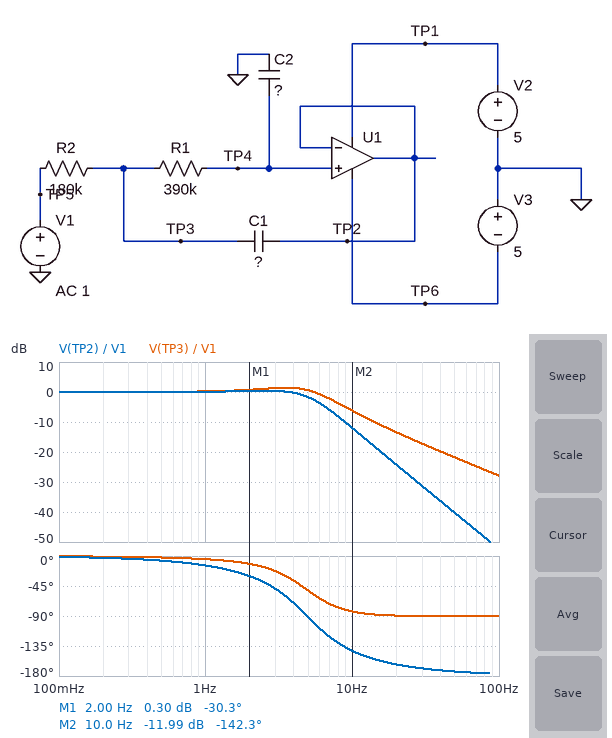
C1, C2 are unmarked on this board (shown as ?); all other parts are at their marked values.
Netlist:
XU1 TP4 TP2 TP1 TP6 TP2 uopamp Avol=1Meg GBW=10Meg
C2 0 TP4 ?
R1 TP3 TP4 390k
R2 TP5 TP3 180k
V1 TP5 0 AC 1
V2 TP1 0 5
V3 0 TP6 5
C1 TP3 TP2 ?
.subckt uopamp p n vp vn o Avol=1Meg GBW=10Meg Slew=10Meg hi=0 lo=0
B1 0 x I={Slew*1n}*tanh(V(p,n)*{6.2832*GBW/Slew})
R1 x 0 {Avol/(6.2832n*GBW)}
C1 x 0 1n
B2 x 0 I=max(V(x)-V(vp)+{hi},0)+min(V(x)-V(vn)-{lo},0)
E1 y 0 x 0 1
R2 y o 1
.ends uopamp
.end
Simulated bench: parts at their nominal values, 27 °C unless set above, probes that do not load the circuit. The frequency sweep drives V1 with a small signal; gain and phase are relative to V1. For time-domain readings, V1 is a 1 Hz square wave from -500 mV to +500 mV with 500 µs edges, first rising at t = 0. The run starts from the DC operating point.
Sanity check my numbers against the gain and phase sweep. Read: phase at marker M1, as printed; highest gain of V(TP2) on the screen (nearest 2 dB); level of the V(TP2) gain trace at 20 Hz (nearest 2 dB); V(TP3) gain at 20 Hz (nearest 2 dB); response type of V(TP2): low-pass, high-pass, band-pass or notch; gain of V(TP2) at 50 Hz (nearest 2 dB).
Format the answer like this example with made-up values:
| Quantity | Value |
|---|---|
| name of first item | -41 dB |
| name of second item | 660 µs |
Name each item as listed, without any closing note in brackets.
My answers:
| Quantity | Value |
|---|---|
| phase at marker M1, as printed | -30.3 deg |
| highest gain of V(TP2) on the screen | 0 dB |
| level of the V(TP2) gain trace at 20 Hz | -24 dB |
| V(TP3) gain at 20 Hz | -14 dB |
| response type of V(TP2): low-pass, high-pass, band-pass or notch | low-pass |
| gain of V(TP2) at 50 Hz | -40 dB |
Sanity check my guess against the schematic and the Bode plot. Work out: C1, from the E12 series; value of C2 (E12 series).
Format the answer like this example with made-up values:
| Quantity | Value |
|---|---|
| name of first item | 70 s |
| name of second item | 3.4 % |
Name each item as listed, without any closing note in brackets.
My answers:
| Quantity | Value |
|---|---|
| C1, from the E12 series | 220 nF |
| value of C2 | 68 nF |
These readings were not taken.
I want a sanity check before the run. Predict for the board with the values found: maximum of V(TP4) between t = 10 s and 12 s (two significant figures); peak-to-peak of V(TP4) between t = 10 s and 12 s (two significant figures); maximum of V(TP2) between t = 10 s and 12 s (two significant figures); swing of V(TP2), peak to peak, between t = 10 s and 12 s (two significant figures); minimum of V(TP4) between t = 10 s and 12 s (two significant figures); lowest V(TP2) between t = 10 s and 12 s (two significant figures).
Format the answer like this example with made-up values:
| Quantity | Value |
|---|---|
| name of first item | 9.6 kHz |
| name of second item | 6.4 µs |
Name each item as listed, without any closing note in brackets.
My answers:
| Quantity | Value |
|---|---|
| maximum of V(TP4) between t = 10 s and 12 s | 600 mV |
| peak-to-peak of V(TP4) between t = 10 s and 12 s | 1.2 V |
| maximum of V(TP2) between t = 10 s and 12 s | 600 mV |
| swing of V(TP2), peak to peak, between t = 10 s and 12 s | 1.2 V |
| minimum of V(TP4) between t = 10 s and 12 s | -600 mV |
| lowest V(TP2) between t = 10 s and 12 s | -600 mV |
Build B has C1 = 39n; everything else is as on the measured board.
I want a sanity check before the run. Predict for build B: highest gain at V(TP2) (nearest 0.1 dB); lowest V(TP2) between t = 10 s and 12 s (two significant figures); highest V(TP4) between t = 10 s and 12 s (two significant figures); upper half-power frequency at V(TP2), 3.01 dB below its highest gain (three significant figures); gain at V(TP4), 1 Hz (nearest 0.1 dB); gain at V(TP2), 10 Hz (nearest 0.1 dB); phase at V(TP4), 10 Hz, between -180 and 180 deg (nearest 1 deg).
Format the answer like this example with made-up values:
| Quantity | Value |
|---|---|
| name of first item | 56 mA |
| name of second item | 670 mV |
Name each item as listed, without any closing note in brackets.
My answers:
| Quantity | Value |
|---|---|
| highest gain at V(TP2) | 0 dB |
| lowest V(TP2) between t = 10 s and 12 s | -500 mV |
| highest V(TP4) between t = 10 s and 12 s | 500 mV |
| upper half-power frequency at V(TP2), 3.01 dB below its highest gain | 4.67 Hz |
| gain at V(TP4), 1 Hz | -0.2 dB |
| gain at V(TP2), 10 Hz | -7.8 dB |
| phase at V(TP4), 10 Hz, between -180 and 180 deg | -84 deg |
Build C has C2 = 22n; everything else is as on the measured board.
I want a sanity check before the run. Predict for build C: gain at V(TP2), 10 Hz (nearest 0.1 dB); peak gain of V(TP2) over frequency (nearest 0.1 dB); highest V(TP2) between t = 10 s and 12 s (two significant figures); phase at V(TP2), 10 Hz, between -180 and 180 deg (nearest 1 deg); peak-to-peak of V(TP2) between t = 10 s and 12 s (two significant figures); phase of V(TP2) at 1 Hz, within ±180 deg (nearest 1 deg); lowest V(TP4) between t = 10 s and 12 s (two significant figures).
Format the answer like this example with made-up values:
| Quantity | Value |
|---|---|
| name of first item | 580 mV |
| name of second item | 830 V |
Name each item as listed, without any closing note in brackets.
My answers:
| Quantity | Value |
|---|---|
| gain at V(TP2), 10 Hz | 1.3 dB |
| peak gain of V(TP2) over frequency | 3.9 dB |
| highest V(TP2) between t = 10 s and 12 s | 820 mV |
| phase at V(TP2), 10 Hz, between -180 and 180 deg | -113 deg |
| peak-to-peak of V(TP2) between t = 10 s and 12 s | 1.6 V |
| phase of V(TP2) at 1 Hz, within ±180 deg | -5 deg |
| lowest V(TP4) between t = 10 s and 12 s | -820 mV |
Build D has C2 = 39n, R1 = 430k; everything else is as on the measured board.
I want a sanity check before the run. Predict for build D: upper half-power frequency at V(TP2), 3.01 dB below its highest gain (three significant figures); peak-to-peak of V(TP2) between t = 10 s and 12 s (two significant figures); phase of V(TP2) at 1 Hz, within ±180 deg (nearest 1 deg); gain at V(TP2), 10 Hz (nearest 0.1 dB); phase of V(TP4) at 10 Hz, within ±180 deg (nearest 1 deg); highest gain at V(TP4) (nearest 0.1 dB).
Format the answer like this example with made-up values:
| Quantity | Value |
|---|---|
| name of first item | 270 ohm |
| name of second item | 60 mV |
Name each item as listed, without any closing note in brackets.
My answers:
| Quantity | Value |
|---|---|
| upper half-power frequency at V(TP2), 3.01 dB below its highest gain | 7.29 Hz |
| peak-to-peak of V(TP2) between t = 10 s and 12 s | 1.4 V |
| phase of V(TP2) at 1 Hz, within ±180 deg | -9 deg |
| gain at V(TP2), 10 Hz | -6.9 dB |
| phase of V(TP4) at 10 Hz, within ±180 deg | -137 deg |
| highest gain at V(TP4) | 1.7 dB |
